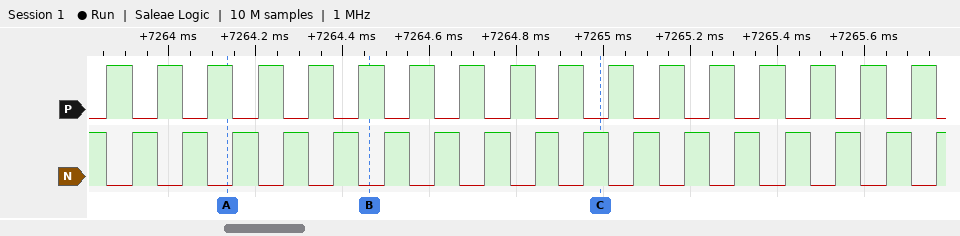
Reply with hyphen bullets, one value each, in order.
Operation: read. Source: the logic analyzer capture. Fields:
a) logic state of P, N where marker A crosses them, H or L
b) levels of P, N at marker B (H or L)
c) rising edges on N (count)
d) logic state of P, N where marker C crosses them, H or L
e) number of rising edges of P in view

- P=H, N=L
- P=H, N=L
- 17
- P=L, N=H
- 17
